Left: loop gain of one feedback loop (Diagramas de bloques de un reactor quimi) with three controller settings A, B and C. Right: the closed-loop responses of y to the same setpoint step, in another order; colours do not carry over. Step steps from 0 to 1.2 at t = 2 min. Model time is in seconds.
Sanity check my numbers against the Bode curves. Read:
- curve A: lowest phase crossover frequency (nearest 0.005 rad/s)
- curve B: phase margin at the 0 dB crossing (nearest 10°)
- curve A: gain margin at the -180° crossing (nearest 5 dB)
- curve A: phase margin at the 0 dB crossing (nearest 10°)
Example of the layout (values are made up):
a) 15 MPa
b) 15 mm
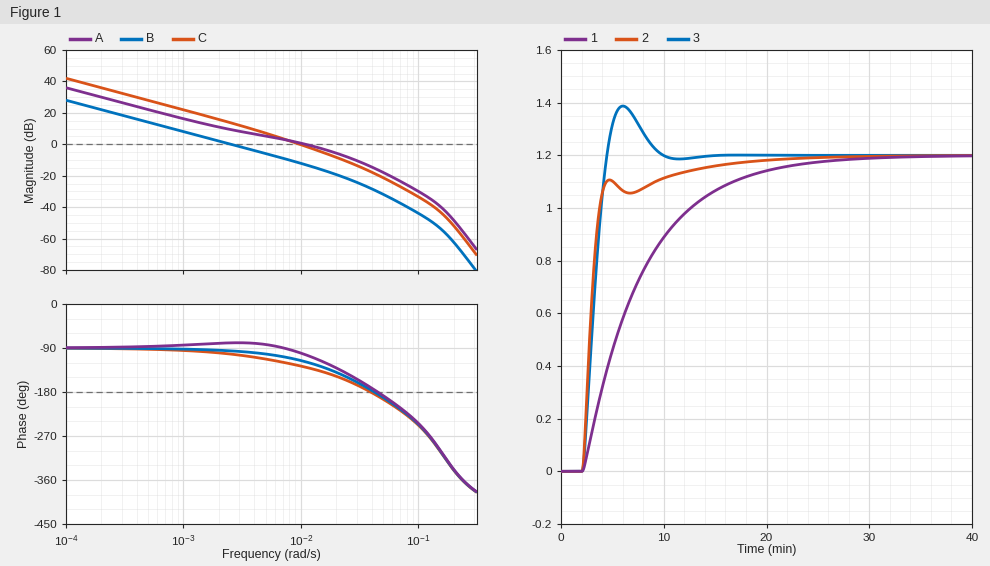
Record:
a) 0.045 rad/s
b) 80°
c) 15 dB
d) 80°
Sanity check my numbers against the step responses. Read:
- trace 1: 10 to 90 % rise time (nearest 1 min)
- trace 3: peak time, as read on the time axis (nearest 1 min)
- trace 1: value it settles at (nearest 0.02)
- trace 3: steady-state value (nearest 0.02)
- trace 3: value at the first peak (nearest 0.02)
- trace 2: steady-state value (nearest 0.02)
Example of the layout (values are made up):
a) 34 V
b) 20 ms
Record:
a) 13 min
b) 6 min
c) 1.20
d) 1.20
e) 1.38
f) 1.20
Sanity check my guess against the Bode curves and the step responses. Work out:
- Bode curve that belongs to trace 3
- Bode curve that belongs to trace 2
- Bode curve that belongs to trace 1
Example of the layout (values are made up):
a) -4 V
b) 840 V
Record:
a) C
b) A
c) B
